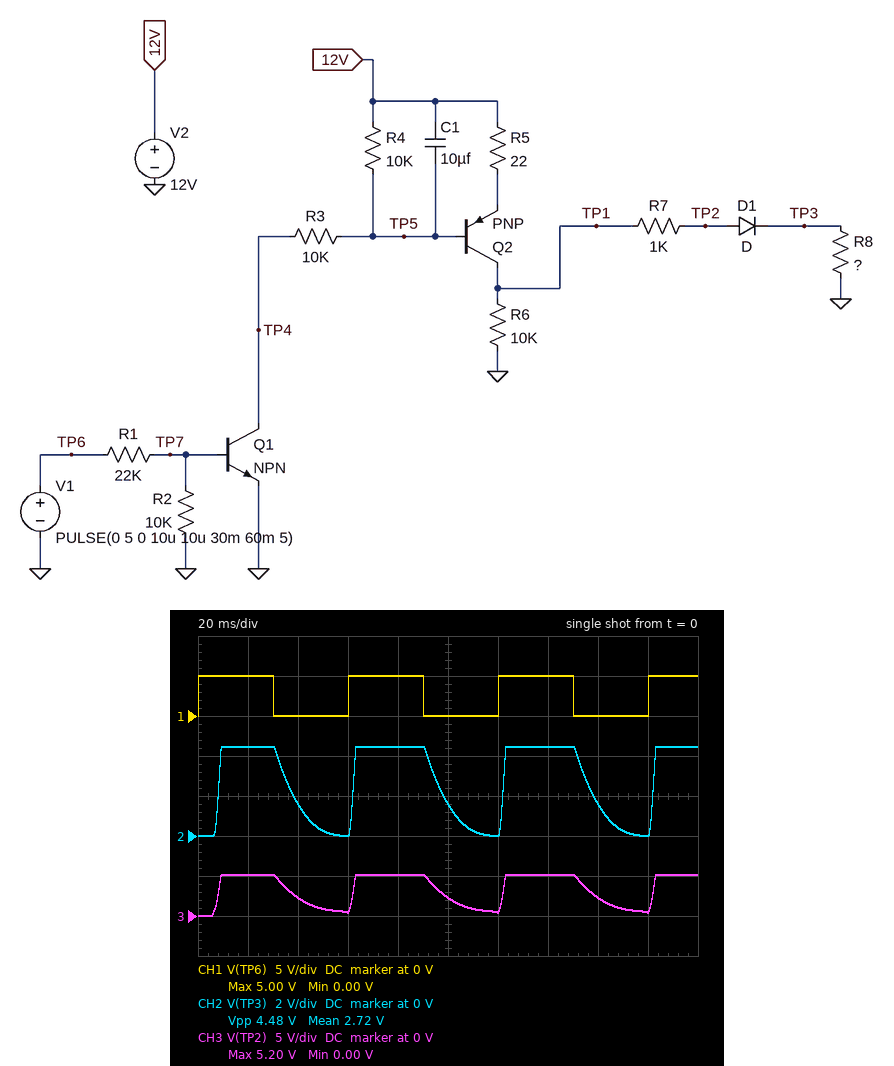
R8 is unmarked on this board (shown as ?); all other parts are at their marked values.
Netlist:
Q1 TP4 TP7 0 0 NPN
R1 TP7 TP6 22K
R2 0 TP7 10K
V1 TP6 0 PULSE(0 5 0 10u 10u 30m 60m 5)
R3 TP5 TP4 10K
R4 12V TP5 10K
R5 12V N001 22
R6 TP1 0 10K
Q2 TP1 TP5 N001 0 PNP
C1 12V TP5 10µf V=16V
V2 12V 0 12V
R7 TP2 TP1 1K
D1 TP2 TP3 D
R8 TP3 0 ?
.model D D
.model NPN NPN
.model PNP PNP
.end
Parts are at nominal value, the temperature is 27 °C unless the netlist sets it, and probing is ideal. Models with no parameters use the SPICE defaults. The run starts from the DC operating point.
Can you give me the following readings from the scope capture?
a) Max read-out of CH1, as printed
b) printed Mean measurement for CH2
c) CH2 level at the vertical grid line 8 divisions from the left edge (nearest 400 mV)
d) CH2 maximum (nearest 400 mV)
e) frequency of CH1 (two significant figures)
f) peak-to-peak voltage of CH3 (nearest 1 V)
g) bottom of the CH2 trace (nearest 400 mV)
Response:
5.00 V
2.72 V
1.6 V
4.4 V
17 Hz
5 V
0 V
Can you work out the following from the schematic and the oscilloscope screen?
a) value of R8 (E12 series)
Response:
680 Ω
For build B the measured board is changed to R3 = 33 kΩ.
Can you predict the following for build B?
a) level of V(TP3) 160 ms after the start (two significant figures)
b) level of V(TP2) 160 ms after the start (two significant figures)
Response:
1.5 V
2.2 V
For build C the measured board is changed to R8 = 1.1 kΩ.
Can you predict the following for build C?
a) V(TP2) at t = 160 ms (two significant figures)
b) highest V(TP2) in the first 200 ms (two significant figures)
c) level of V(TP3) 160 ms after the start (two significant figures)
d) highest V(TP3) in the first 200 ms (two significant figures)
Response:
2.6 V
6.5 V
1.9 V
5.8 V
